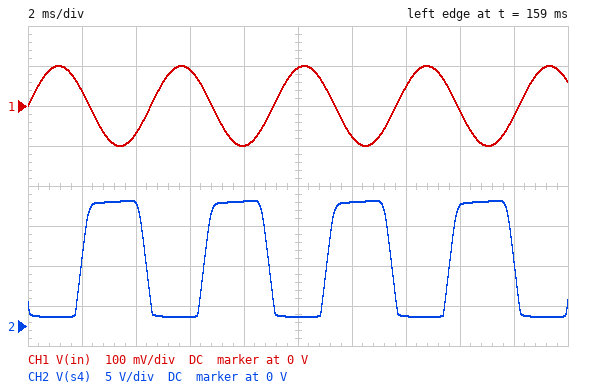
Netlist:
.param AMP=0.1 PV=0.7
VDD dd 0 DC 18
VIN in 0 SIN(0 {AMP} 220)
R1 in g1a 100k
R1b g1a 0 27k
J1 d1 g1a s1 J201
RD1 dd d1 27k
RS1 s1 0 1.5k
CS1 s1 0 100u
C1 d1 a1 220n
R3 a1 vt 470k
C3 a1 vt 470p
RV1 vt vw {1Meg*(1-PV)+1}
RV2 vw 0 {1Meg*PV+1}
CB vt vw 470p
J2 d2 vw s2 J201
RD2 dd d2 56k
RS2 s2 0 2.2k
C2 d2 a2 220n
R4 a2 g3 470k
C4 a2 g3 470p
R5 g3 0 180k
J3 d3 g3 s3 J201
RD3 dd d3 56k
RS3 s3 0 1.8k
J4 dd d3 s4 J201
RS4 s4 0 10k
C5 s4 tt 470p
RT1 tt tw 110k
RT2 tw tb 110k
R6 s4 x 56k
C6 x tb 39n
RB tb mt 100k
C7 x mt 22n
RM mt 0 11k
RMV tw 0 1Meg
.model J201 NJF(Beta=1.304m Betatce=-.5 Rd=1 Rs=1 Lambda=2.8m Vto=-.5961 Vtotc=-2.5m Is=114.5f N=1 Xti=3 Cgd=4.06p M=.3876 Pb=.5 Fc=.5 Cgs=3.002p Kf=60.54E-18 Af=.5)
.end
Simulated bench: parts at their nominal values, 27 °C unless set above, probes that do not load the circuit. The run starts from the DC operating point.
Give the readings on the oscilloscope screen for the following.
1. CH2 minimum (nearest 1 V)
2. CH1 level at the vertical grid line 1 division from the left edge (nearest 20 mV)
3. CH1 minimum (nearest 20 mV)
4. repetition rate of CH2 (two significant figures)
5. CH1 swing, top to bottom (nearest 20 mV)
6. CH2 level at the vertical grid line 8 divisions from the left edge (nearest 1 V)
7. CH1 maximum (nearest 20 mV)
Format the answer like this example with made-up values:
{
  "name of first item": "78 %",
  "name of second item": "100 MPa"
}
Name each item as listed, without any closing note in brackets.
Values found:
{
  "CH2 minimum": "1 V",
  "CH1 level at the vertical grid line 1 division from the left edge": "40 mV",
  "CH1 minimum": "-100 mV",
  "repetition rate of CH2": "220 Hz",
  "CH1 swing, top to bottom": "200 mV",
  "CH2 level at the vertical grid line 8 divisions from the left edge": "15 V",
  "CH1 maximum": "100 mV"
}
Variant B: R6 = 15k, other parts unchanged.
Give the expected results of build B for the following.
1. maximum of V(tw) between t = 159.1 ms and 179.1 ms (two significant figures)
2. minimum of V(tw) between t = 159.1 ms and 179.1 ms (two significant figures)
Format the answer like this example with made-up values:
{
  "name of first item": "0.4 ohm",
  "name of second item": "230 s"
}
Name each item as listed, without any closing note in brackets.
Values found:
{
  "maximum of V(tw) between t = 159.1 ms and 179.1 ms": "5.1 V",
  "minimum of V(tw) between t = 159.1 ms and 179.1 ms": "-5.4 V"
}
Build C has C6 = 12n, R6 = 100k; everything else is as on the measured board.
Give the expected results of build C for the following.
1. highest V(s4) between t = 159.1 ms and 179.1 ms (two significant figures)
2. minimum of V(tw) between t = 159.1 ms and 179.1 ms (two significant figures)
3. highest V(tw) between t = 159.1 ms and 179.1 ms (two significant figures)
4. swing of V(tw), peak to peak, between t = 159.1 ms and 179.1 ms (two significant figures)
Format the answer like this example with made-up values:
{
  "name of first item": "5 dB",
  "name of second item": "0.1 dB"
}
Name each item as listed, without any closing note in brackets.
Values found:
{
  "highest V(s4) between t = 159.1 ms and 179.1 ms": "16 V",
  "minimum of V(tw) between t = 159.1 ms and 179.1 ms": "-2.0 V",
  "highest V(tw) between t = 159.1 ms and 179.1 ms": "1.9 V",
  "swing of V(tw), peak to peak, between t = 159.1 ms and 179.1 ms": "3.8 V"
}
